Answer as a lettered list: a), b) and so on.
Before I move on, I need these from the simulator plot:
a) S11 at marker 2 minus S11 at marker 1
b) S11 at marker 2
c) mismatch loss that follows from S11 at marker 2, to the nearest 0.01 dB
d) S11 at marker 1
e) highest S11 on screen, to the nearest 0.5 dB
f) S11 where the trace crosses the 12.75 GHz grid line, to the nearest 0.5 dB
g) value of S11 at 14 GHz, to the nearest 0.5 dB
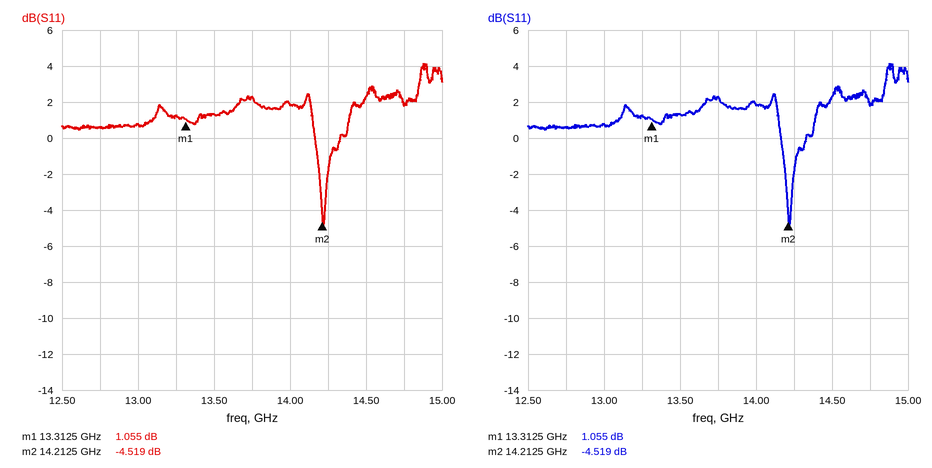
a) -5.574 dB
b) -4.519 dB
c) 1.89 dB
d) 1.055 dB
e) 4.0 dB
f) 0.5 dB
g) 2.0 dB
